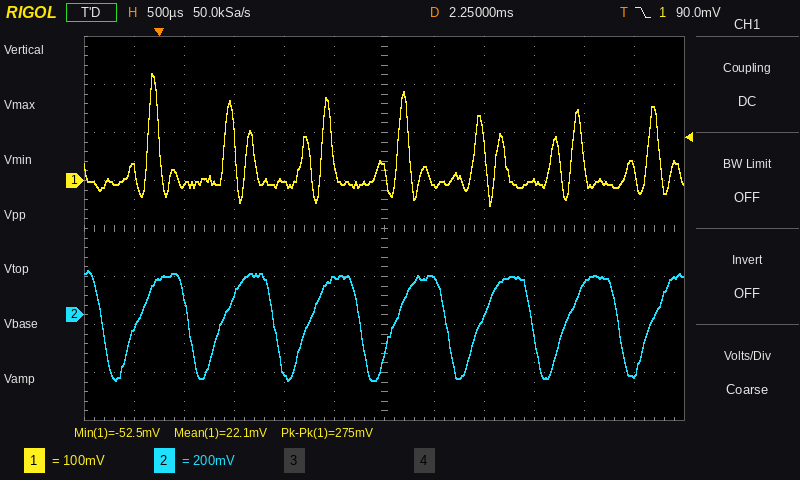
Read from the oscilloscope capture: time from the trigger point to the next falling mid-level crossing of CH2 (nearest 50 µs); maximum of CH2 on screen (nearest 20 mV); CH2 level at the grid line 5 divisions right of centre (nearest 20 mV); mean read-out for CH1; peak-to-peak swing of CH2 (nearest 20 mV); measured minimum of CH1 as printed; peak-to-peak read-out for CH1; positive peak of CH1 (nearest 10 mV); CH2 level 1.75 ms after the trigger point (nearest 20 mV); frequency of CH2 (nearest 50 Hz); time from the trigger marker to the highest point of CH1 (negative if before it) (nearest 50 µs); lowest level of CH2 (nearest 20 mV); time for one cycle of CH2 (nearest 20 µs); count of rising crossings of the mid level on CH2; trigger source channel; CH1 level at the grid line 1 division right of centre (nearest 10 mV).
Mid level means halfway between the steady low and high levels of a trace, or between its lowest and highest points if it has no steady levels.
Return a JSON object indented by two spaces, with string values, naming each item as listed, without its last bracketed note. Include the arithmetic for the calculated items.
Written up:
{
  "time from the trigger point to the next falling mid-level crossing of CH2": "300 µs",
  "maximum of CH2 on screen": "180 mV",
  "CH2 level at the grid line 5 divisions right of centre": "-240 mV",
  "mean read-out for CH1": "22.1 mV",
  "peak-to-peak swing of CH2": "180 mV − (-280 mV) = 460 mV",
  "measured minimum of CH1 as printed": "-52.5 mV",
  "peak-to-peak read-out for CH1": "275 mV",
  "positive peak of CH1": "220 mV",
  "CH2 level 1.75 ms after the trigger point": "160 mV",
  "frequency of CH2": "1 / 860 µs ≈ 1.16 kHz, so 1.15 kHz to the nearest 50 Hz",
  "time from the trigger marker to the highest point of CH1 (negative if before it)": "-50 µs",
  "lowest level of CH2": "-280 mV",
  "time for one cycle of CH2": "860 µs",
  "count of rising crossings of the mid level on CH2": "7",
  "trigger source channel": "CH1",
  "CH1 level at the grid line 1 division right of centre": "-10 mV"
}
